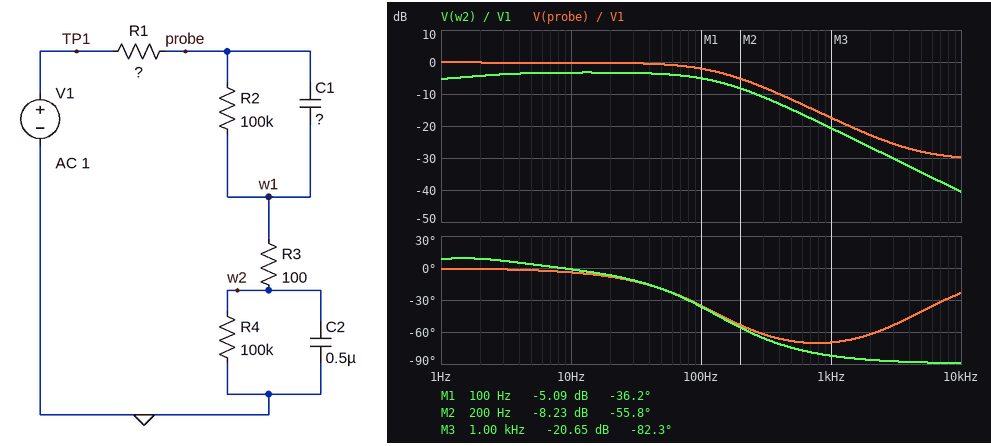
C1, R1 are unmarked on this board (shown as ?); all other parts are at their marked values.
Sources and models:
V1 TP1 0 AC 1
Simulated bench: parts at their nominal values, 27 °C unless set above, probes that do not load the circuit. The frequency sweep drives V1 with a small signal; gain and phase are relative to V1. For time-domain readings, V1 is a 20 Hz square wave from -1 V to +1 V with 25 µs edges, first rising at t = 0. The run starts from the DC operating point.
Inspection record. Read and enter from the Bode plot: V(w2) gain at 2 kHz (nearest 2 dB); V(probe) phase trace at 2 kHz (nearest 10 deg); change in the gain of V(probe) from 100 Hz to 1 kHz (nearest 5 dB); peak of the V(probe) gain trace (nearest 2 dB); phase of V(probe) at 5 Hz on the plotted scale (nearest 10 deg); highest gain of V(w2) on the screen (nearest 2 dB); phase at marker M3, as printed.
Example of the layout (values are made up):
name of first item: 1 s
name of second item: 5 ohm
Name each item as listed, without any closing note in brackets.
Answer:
V(w2) gain at 2 kHz: -26 dB
V(probe) phase trace at 2 kHz: -60 deg
change in the gain of V(probe) from 100 Hz to 1 kHz: -15 dB
peak of the V(probe) gain trace: 0 dB
phase of V(probe) at 5 Hz on the plotted scale: 0 deg
highest gain of V(w2) on the screen: -4 dB
phase at marker M3, as printed: -82.3 deg
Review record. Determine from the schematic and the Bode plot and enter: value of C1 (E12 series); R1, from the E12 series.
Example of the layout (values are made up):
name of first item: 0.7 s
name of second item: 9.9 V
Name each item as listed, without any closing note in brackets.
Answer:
value of C1: 1.2 µF
R1, from the E12 series: 3.3 kΩ
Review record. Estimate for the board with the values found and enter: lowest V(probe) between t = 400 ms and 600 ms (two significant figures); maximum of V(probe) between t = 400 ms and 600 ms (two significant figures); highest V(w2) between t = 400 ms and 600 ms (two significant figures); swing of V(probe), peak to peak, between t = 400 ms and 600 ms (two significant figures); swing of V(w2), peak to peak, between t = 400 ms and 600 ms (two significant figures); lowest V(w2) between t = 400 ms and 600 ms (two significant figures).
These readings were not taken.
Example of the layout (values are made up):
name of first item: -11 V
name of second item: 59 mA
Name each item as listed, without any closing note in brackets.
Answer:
lowest V(probe) between t = 400 ms and 600 ms: -980 mV
maximum of V(probe) between t = 400 ms and 600 ms: 980 mV
highest V(w2) between t = 400 ms and 600 ms: 700 mV
swing of V(probe), peak to peak, between t = 400 ms and 600 ms: 2.0 V
swing of V(w2), peak to peak, between t = 400 ms and 600 ms: 1.4 V
lowest V(w2) between t = 400 ms and 600 ms: -700 mV
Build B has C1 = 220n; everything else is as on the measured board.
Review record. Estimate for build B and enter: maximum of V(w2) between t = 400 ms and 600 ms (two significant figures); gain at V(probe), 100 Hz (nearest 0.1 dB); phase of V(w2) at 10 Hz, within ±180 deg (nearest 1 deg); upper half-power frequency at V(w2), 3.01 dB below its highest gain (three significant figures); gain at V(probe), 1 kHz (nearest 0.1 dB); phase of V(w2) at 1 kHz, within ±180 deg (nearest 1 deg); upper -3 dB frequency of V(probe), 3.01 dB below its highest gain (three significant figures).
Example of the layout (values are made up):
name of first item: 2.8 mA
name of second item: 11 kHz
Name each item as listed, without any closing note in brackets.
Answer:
maximum of V(w2) between t = 400 ms and 600 ms: 360 mV
gain at V(probe), 100 Hz: -0.6 dB
phase of V(w2) at 10 Hz, within ±180 deg: -14 deg
upper half-power frequency at V(w2), 3.01 dB below its highest gain: 8.68 Hz
gain at V(probe), 1 kHz: -10.6 dB
phase of V(w2) at 1 kHz, within ±180 deg: -73 deg
upper -3 dB frequency of V(probe), 3.01 dB below its highest gain: 311 Hz
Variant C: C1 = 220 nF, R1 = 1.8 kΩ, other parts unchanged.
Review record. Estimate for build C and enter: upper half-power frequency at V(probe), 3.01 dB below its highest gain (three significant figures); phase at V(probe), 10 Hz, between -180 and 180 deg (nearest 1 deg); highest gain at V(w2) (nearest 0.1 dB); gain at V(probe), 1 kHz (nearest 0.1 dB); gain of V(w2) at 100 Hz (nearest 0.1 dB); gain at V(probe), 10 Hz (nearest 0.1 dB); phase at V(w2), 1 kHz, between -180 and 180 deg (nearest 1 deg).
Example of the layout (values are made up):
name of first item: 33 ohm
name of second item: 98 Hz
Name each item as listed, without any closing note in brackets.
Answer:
upper half-power frequency at V(probe), 3.01 dB below its highest gain: 554 Hz
phase at V(probe), 10 Hz, between -180 and 180 deg: -1 deg
highest gain at V(w2): -6.1 dB
gain at V(probe), 1 kHz: -6.3 dB
gain of V(w2) at 100 Hz: -10.5 dB
gain at V(probe), 10 Hz: -0.1 dB
phase at V(w2), 1 kHz, between -180 and 180 deg: -61 deg
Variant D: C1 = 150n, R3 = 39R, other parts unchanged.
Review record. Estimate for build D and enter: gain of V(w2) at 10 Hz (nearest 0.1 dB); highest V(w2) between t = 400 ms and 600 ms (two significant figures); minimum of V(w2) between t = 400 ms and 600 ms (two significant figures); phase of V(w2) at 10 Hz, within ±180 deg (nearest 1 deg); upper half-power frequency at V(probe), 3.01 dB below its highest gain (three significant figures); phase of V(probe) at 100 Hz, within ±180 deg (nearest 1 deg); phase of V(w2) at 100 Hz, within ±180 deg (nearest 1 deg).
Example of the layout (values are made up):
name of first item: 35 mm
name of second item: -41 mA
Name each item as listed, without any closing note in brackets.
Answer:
gain of V(w2) at 10 Hz: -10.6 dB
highest V(w2) between t = 400 ms and 600 ms: 320 mV
minimum of V(w2) between t = 400 ms and 600 ms: -320 mV
phase of V(w2) at 10 Hz, within ±180 deg: -22 deg
upper half-power frequency at V(probe), 3.01 dB below its highest gain: 418 Hz
phase of V(probe) at 100 Hz, within ±180 deg: -13 deg
phase of V(w2) at 100 Hz, within ±180 deg: -17 deg
